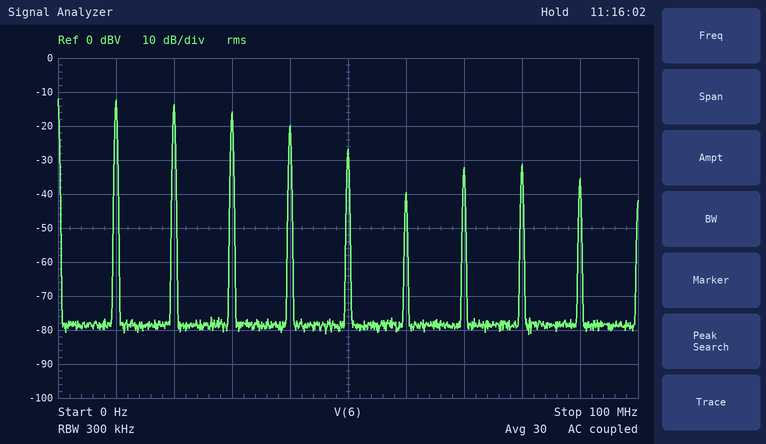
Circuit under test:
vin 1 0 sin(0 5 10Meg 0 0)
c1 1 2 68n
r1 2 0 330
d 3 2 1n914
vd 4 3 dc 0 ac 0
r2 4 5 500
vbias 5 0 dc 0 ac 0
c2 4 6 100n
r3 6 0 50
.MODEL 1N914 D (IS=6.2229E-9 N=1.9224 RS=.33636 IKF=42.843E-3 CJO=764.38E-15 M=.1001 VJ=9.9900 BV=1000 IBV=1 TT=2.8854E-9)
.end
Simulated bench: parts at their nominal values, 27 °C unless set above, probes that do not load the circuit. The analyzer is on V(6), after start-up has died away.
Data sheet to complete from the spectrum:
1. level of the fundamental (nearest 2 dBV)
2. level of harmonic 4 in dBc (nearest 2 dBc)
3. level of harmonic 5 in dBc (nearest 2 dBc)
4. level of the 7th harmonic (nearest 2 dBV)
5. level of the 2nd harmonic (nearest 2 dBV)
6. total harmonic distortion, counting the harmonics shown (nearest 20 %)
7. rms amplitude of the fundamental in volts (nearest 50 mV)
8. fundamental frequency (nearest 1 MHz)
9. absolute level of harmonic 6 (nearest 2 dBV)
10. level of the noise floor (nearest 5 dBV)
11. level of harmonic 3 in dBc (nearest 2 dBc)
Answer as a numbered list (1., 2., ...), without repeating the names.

1. -12 dBV
2. -8 dBc
3. -14 dBc
4. -32 dBV
5. -14 dBV
6. 120 %
7. 250 mV
8. 10 MHz
9. -40 dBV
10. -80 dBV
11. -4 dBc
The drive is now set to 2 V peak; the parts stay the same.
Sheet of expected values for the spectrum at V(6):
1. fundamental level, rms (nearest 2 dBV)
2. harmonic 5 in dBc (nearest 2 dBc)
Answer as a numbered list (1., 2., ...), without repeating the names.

1. -22 dBV
2. -12 dBc
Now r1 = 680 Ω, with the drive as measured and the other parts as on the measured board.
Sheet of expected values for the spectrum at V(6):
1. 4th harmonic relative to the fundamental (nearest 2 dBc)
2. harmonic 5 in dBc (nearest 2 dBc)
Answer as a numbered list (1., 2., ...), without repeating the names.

1. -6 dBc
2. -10 dBc
